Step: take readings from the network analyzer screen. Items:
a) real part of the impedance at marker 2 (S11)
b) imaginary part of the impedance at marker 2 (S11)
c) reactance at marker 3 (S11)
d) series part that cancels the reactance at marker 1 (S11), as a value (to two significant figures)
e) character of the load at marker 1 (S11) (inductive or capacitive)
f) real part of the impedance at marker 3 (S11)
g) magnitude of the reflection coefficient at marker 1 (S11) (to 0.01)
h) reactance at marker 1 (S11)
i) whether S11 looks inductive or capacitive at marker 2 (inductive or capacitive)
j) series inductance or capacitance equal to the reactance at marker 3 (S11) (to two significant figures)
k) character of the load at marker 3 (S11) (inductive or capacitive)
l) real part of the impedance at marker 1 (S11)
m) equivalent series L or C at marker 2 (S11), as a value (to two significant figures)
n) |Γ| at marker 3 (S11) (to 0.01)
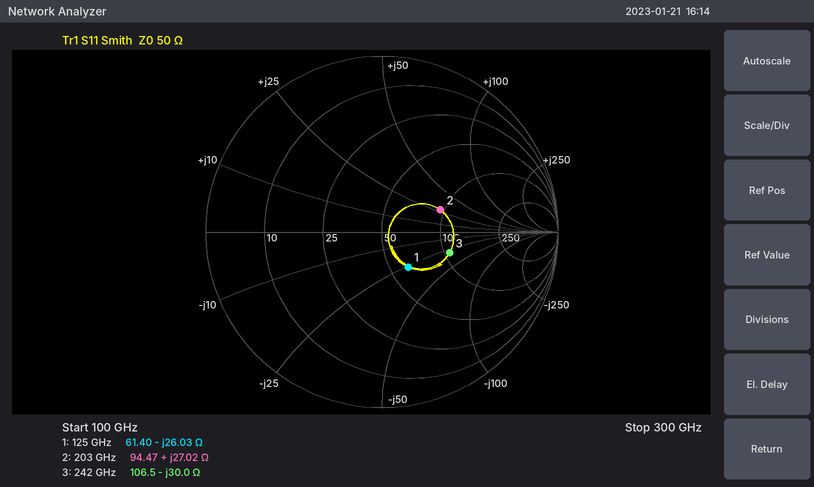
94.47 Ω
+27.02 Ω
-30.0 Ω
33 pH
capacitive
106.5 Ω
0.25
-26.03 Ω
inductive
22 fF
capacitive
61.40 Ω
21 pH
0.40
